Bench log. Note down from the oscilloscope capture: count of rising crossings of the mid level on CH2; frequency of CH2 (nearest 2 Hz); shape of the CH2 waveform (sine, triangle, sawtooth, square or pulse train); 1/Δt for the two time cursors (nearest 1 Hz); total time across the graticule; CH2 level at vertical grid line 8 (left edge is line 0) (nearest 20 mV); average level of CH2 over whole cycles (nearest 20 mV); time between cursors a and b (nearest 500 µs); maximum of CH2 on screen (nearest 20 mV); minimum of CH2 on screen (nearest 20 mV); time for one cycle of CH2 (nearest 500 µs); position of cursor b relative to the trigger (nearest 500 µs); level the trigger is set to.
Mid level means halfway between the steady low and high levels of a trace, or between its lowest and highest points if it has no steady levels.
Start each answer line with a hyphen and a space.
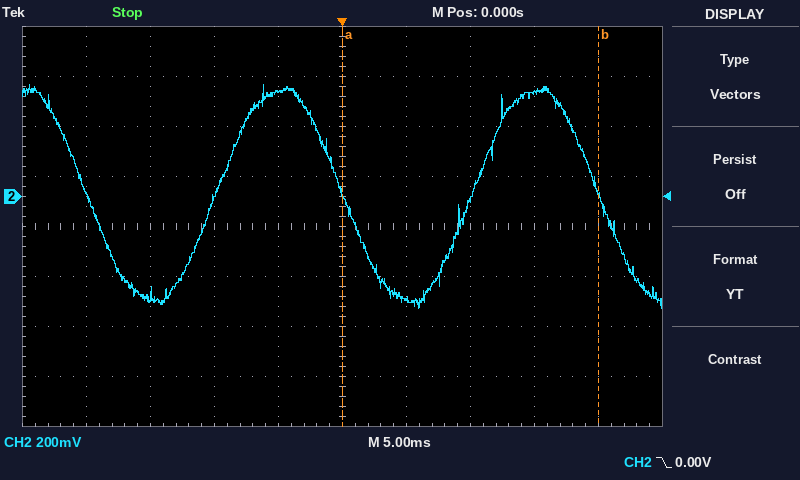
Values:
- 2
- 50 Hz
- sine
- 50 Hz
- 50 ms
- 420 mV
- 0 mV
- 20.0 ms
- 440 mV
- -440 mV
- 20.0 ms
- +20.0 ms
- 0.00 V
